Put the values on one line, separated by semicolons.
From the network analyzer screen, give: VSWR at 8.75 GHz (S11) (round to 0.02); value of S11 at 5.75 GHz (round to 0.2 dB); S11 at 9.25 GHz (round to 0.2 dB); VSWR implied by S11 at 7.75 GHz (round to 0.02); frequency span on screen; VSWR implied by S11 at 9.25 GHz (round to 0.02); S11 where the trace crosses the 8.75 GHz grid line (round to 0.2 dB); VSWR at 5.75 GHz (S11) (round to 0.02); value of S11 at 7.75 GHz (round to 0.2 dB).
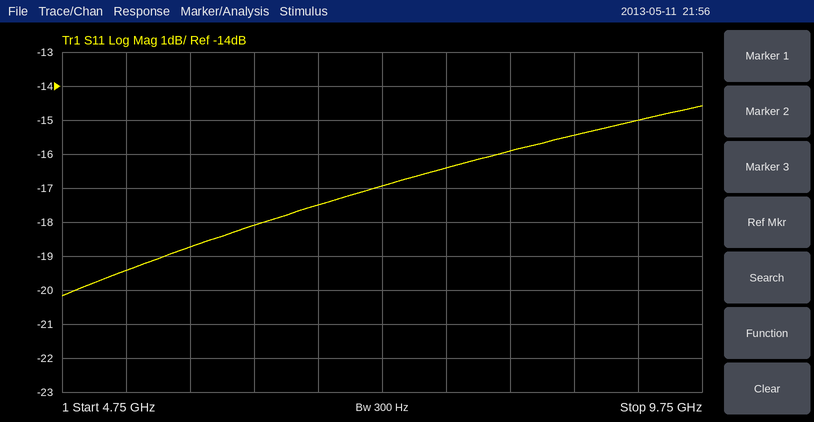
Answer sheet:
1.40; -18.8 dB; -15.0 dB; 1.36; 5 GHz; 1.44; -15.4 dB; 1.26; -16.4 dB
